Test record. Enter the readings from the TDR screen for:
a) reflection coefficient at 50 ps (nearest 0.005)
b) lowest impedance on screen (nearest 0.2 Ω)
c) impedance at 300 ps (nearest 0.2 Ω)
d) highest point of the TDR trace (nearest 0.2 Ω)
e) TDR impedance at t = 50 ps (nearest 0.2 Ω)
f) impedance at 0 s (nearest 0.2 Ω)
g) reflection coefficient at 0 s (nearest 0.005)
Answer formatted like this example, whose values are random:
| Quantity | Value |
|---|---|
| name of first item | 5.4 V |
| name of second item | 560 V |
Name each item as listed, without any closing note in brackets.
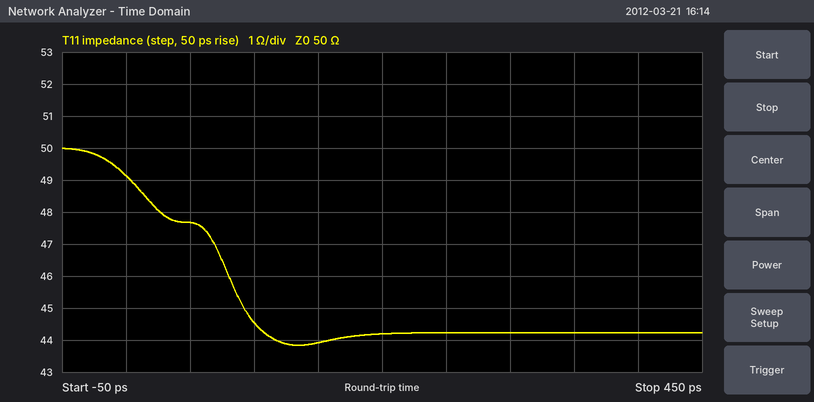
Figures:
| Quantity | Value |
|---|---|
| reflection coefficient at 50 ps | -0.025 |
| lowest impedance on screen | 43.8 Ω |
| impedance at 300 ps | 44.2 Ω |
| highest point of the TDR trace | 50.0 Ω |
| TDR impedance at t = 50 ps | 47.6 Ω |
| impedance at 0 s | 49.2 Ω |
| reflection coefficient at 0 s | -0.010 |
